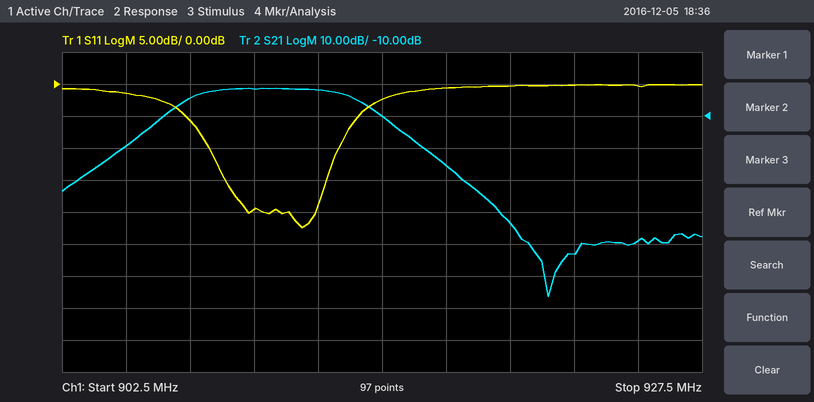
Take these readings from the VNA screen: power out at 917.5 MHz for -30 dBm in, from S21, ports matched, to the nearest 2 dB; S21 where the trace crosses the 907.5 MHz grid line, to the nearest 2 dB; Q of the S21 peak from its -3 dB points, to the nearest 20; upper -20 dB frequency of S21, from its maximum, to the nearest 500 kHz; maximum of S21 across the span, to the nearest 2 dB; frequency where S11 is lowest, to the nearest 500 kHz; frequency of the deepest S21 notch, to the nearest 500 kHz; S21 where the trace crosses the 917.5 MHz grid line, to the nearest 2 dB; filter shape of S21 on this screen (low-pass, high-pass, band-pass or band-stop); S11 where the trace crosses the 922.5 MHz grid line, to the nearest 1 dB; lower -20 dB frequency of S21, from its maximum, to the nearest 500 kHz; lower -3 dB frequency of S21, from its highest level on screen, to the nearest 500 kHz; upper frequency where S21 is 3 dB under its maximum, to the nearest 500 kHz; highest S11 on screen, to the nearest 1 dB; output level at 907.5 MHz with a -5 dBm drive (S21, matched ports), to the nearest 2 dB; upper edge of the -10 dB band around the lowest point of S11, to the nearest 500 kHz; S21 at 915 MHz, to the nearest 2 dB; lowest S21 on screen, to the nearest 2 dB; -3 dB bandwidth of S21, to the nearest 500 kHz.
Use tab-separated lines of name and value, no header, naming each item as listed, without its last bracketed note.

power out at 917.5 MHz for -30 dBm in, from S21, ports matched, to the nearest 2 dB	-56 dBm
S21 where the trace crosses the 907.5 MHz grid line, to the nearest 2 dB	-4 dB
Q of the S21 peak from its -3 dB points, to the nearest 20	140
upper -20 dB frequency of S21, from its maximum, to the nearest 500 kHz	917.0 MHz
maximum of S21 across the span, to the nearest 2 dB	-2 dB
frequency where S11 is lowest, to the nearest 500 kHz	912.0 MHz
frequency of the deepest S21 notch, to the nearest 500 kHz	921.5 MHz
S21 where the trace crosses the 917.5 MHz grid line, to the nearest 2 dB	-26 dB
filter shape of S21 on this screen	band-pass
S11 where the trace crosses the 922.5 MHz grid line, to the nearest 1 dB	0 dB
lower -20 dB frequency of S21, from its maximum, to the nearest 500 kHz	904.5 MHz
lower -3 dB frequency of S21, from its highest level on screen, to the nearest 500 kHz	907.5 MHz
upper frequency where S21 is 3 dB under its maximum, to the nearest 500 kHz	914.0 MHz
highest S11 on screen, to the nearest 1 dB	0 dB
output level at 907.5 MHz with a -5 dBm drive (S21, matched ports), to the nearest 2 dB	-10 dBm
upper edge of the -10 dB band around the lowest point of S11, to the nearest 500 kHz	913.5 MHz
S21 at 915 MHz, to the nearest 2 dB	-10 dB
lowest S21 on screen, to the nearest 2 dB	-66 dB
-3 dB bandwidth of S21, to the nearest 500 kHz	6.5 MHz
